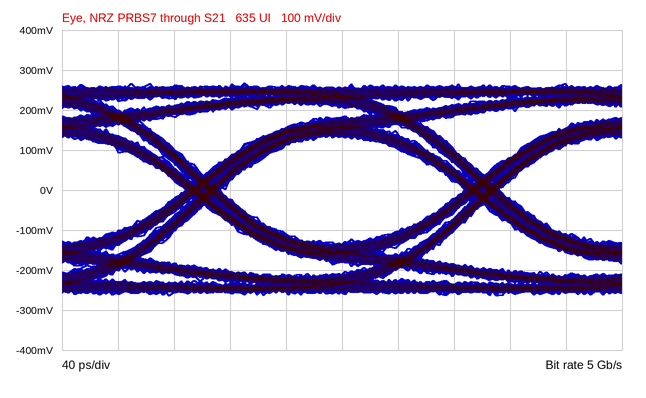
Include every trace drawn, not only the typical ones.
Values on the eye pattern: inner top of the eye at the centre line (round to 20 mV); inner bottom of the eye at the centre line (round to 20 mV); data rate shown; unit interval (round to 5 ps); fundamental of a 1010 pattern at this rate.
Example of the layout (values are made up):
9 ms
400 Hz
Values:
140 mV
-140 mV
5 Gb/s
200 ps
2.5 GHz
